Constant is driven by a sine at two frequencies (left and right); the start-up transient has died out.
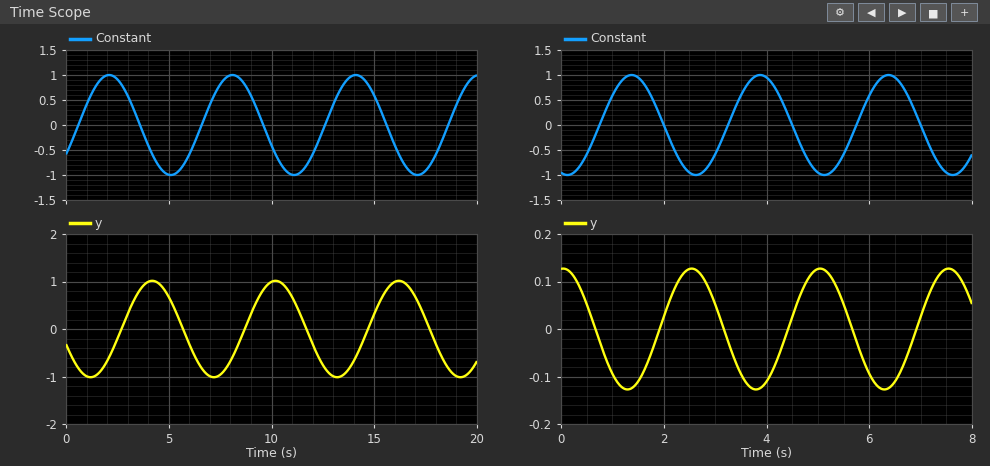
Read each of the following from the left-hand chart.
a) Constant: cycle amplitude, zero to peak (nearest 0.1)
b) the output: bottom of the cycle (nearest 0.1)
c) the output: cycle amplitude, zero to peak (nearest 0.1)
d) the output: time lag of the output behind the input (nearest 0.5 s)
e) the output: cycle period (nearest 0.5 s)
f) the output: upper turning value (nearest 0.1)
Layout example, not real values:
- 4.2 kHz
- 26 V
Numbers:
- 1.0
- -1.0
- 1.0
- 2.0 s
- 6.0 s
- 1.0
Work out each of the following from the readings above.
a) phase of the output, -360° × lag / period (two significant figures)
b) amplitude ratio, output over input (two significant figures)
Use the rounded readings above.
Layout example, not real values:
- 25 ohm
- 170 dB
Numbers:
- -120°
- 1.0
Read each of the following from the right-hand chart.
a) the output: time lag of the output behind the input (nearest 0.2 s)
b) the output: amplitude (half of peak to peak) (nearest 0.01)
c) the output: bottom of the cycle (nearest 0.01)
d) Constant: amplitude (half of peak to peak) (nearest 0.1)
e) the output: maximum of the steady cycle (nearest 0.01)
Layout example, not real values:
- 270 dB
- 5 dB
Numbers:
- 1.2 s
- 0.13
- -0.13
- 1.0
- 0.13
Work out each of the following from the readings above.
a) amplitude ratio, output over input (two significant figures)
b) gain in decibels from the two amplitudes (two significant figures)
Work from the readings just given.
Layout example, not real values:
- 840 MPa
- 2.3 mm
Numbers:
- 0.13
- -18 dB
